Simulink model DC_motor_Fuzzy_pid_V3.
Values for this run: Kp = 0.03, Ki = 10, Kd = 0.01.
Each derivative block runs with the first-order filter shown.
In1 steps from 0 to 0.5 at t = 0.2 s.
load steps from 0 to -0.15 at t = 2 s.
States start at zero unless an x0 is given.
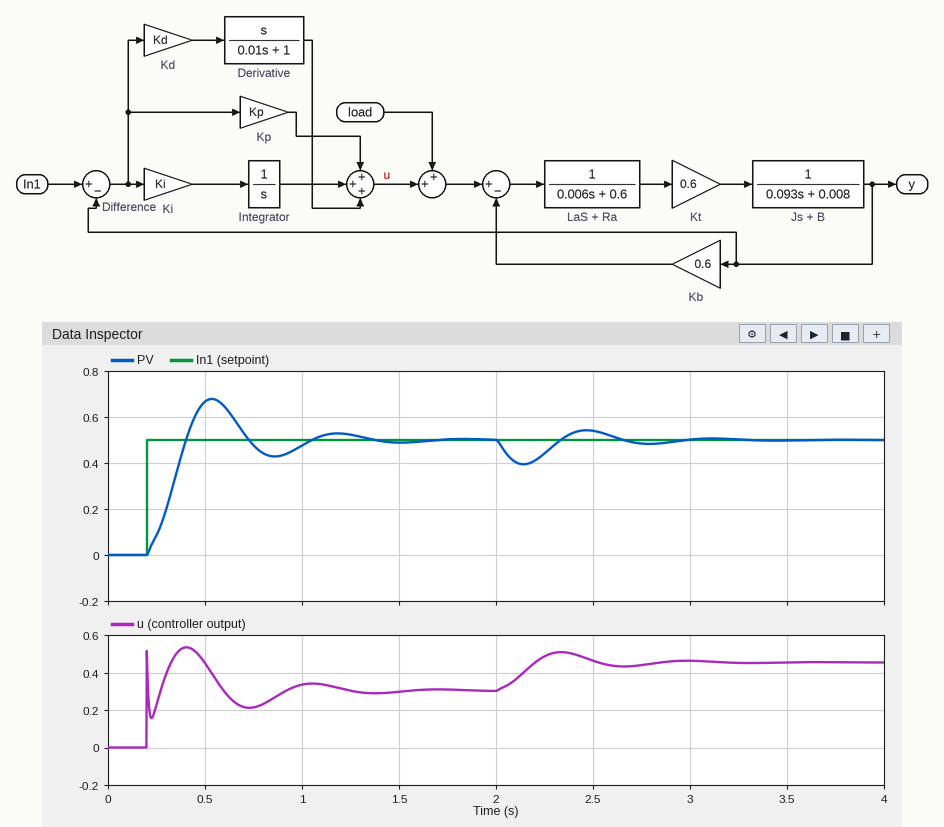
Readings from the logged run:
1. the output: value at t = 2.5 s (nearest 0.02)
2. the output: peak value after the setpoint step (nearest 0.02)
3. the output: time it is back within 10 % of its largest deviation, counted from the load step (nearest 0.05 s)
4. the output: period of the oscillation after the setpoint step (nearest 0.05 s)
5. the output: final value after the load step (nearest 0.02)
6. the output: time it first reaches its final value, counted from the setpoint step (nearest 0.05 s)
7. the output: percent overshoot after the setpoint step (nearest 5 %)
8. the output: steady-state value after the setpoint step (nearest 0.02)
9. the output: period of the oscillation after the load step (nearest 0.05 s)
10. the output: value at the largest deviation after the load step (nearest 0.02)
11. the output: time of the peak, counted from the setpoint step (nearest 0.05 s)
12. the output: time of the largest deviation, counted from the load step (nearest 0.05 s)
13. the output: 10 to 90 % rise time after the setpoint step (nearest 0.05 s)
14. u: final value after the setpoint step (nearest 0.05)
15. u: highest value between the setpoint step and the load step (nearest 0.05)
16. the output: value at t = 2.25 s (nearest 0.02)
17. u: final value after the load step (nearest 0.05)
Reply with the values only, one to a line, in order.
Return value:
0.54
0.68
0.90 s
0.65 s
0.50
0.20 s
35 %
0.50
0.65 s
0.40
0.35 s
0.15 s
0.15 s
0.30
0.55
0.44
0.45
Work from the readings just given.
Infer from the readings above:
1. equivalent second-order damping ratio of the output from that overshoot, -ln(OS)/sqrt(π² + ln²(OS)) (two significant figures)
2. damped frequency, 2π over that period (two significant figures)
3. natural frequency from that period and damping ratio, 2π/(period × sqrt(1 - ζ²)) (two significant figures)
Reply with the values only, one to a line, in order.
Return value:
0.32
9.7 rad/s
10 rad/s
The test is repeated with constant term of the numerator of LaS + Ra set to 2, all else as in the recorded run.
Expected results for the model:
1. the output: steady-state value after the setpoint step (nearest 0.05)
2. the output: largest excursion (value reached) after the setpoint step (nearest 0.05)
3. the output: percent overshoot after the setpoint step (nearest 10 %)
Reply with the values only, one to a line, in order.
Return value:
0.50
0.60
20 %
